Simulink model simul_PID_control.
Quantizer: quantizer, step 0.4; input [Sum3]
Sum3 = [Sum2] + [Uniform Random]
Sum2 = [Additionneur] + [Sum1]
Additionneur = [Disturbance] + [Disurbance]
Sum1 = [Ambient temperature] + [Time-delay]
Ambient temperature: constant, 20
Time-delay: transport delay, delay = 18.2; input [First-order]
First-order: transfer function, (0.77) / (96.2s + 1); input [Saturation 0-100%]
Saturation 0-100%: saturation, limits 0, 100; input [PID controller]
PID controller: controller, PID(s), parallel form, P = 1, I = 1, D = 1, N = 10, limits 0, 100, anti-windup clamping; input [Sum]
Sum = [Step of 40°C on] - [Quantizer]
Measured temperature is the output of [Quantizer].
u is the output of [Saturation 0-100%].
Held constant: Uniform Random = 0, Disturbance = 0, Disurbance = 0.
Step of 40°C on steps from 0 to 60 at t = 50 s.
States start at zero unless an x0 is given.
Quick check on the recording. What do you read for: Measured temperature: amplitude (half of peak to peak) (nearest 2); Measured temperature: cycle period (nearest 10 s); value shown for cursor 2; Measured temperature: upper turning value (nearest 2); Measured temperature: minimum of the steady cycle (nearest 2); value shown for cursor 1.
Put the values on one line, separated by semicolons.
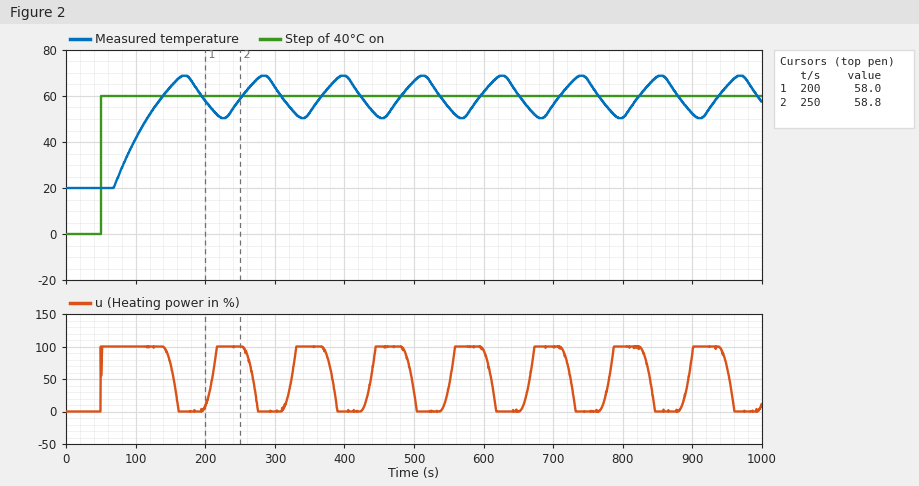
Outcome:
10; 110 s; 58.8; 68; 50; 58.0
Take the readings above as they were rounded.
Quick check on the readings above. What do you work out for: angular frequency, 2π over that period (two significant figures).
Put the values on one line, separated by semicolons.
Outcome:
0.057 rad/s
